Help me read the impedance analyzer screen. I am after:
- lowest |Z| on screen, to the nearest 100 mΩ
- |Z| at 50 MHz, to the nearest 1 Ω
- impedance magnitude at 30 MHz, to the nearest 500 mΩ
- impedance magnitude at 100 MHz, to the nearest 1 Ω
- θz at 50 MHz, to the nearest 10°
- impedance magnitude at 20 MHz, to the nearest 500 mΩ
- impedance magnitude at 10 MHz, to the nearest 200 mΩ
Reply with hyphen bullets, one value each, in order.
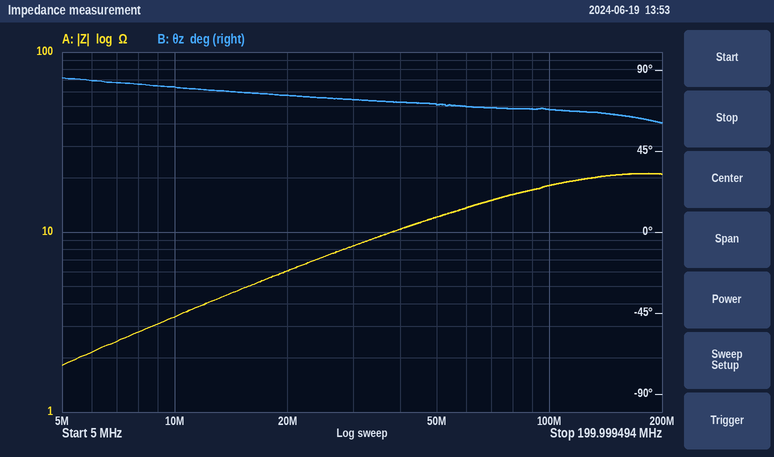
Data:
- 1.8 Ω
- 12 Ω
- 8.5 Ω
- 18 Ω
- 70°
- 6.0 Ω
- 3.4 Ω
